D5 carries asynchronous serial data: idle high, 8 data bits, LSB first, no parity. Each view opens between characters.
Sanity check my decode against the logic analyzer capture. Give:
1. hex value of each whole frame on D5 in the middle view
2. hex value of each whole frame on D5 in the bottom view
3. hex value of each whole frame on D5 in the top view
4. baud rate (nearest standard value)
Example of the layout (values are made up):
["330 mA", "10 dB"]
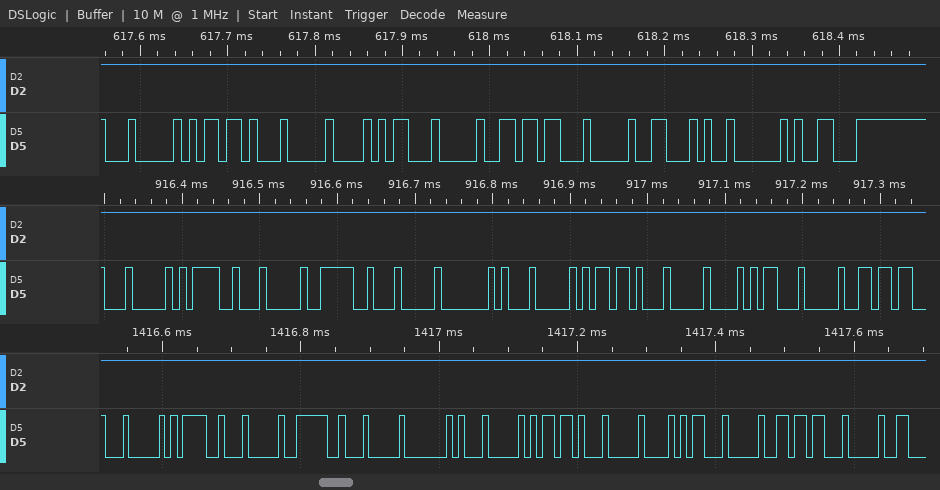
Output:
["04, 3D, 04, 3E, 04, 40, 04, 6D, 04, A8, 04, B6", "04, 3D, 04, 3E, 04, 40, 04, 6D, 04, A8, 04, B6, 04", "04, 6D, 04, A8, 04, B6, 04, 46, 02, 19", "115200 baud"]
